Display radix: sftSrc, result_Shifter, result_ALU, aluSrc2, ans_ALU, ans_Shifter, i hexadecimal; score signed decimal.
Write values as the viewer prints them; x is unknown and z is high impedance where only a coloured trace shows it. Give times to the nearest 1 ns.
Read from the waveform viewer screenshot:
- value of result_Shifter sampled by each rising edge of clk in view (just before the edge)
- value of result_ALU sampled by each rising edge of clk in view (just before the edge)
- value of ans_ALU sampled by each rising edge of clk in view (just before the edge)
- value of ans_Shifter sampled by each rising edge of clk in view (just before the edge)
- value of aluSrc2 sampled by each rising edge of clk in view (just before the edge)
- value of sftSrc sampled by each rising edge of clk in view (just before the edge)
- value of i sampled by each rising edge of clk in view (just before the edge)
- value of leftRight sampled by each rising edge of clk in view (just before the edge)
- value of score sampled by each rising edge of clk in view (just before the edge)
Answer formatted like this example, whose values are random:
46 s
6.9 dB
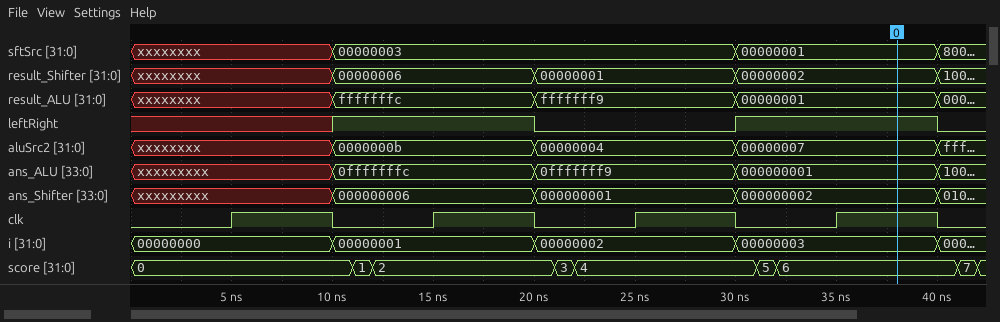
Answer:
xxxxxxxx, 00000006, 00000001, 00000002
xxxxxxxx, fffffffc, fffffff9, 00000001
xxxxxxxxx, 0fffffffc, 0fffffff9, 000000001
xxxxxxxxx, 000000006, 000000001, 000000002
xxxxxxxx, 0000000b, 00000004, 00000007
xxxxxxxx, 00000003, 00000003, 00000001
00000000, 00000001, 00000002, 00000003
x 1 0 1
0, 2, 4, 6
